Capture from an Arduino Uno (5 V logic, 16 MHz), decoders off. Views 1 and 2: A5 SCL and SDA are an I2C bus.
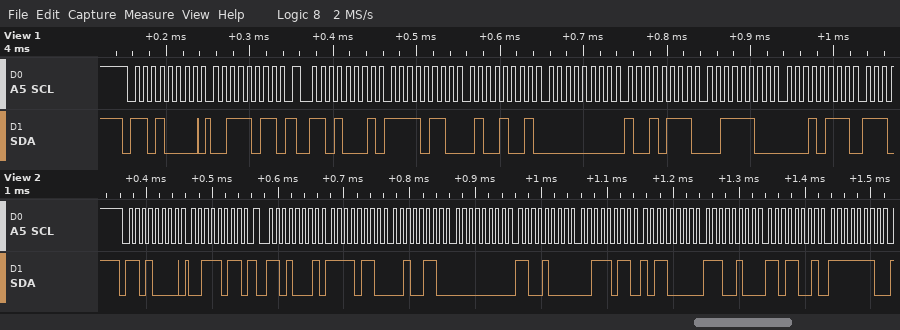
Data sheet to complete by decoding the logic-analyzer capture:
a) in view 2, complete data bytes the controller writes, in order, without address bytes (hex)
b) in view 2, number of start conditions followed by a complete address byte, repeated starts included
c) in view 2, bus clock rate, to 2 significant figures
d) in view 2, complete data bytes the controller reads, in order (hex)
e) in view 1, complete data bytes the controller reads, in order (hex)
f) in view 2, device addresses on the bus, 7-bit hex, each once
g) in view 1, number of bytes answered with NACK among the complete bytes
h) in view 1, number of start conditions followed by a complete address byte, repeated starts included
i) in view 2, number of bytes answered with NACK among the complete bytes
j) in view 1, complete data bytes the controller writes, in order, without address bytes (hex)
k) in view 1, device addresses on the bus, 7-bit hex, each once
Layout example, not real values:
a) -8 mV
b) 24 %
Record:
a) 3B
b) 2
c) 100 kHz
d) F6 26 00 C8 3B B0 E4 D9 FE
e) F6 49 00 97 3C 17
f) 0x68
g) 0
h) 2
i) 0
j) 3B
k) 0x68
